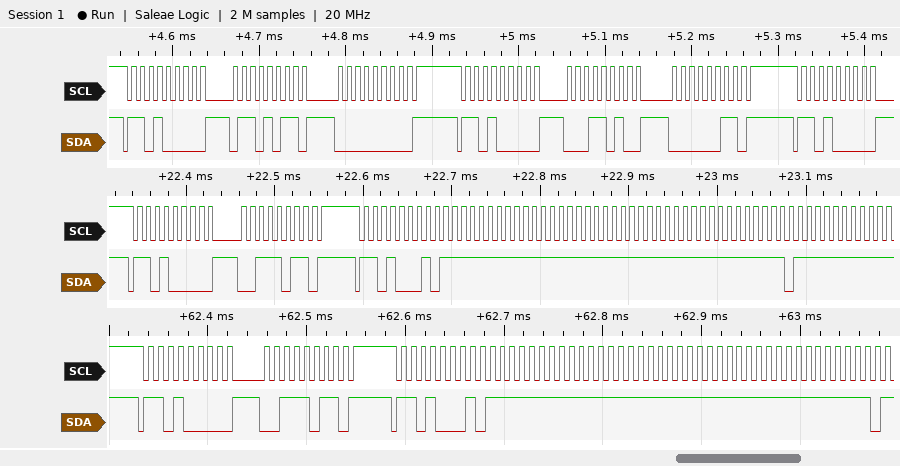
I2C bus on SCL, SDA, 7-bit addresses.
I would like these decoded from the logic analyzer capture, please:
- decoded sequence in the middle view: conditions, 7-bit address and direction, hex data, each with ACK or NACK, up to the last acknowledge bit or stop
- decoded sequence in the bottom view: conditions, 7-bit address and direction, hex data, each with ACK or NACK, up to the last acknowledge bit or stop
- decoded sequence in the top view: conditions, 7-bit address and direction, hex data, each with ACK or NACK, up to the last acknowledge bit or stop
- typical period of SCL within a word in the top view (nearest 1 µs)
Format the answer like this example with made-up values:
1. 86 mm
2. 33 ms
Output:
1. start, address 68 write ACK, 3B ACK, repeated start, address 68 read ACK, FF NACK, FF NACK, FF NACK, FF NACK, EF NACK
2. start, address 68 write ACK, 3B ACK, repeated start, address 68 read ACK, FF NACK, FF NACK, FF NACK, FF NACK
3. start, address 68 write ACK, 6B ACK, 00 ACK, repeated start, address 68 write ACK, 1A ACK, 03 ACK, repeated start, address 68 write ACK
4. 10 µs
